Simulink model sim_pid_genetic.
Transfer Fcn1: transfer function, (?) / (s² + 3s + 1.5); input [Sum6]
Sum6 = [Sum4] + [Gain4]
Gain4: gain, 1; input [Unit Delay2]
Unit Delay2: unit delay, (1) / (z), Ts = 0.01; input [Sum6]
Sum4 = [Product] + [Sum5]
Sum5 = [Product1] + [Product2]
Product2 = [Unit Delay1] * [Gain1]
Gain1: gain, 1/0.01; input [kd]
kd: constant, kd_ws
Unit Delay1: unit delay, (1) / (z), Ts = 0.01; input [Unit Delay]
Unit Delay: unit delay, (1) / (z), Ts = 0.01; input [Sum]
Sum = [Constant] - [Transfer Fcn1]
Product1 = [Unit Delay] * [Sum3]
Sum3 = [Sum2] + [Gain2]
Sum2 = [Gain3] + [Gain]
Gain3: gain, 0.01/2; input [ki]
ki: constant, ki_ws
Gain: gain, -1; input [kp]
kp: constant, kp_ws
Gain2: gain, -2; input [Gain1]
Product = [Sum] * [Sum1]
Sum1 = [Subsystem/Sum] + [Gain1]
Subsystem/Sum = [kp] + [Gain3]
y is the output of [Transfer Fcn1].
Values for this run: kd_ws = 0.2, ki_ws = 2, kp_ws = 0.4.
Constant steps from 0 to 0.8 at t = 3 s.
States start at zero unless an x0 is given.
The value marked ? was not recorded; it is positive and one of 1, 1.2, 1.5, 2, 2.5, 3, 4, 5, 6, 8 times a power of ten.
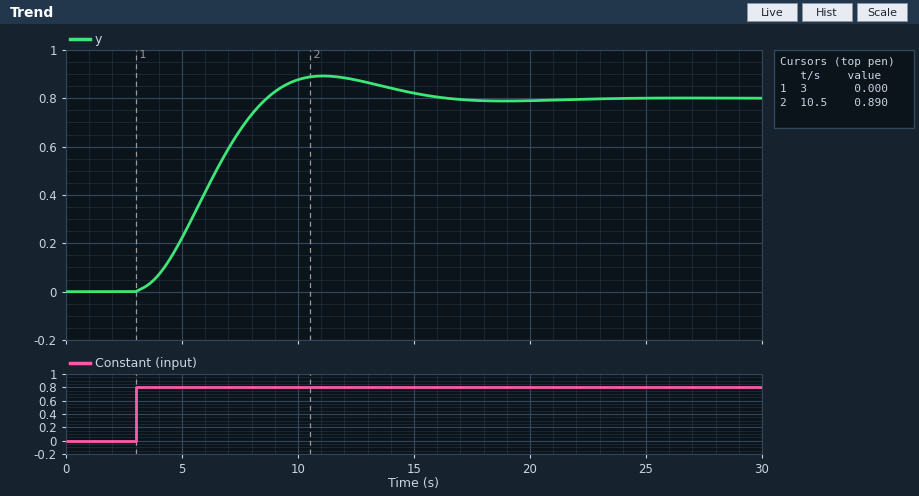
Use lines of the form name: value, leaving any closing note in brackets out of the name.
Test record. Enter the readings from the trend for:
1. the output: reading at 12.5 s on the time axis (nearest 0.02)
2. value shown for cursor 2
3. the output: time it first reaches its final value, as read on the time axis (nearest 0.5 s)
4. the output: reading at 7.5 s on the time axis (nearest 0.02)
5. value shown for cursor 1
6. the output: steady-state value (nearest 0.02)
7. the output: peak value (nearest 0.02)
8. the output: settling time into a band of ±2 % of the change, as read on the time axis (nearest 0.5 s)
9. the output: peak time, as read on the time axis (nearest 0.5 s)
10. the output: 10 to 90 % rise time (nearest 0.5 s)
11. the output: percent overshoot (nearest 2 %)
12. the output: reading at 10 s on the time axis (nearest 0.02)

the output: reading at 12.5 s on the time axis: 0.88
value shown for cursor 2: 0.890
the output: time it first reaches its final value, as read on the time axis: 8.5 s
the output: reading at 7.5 s on the time axis: 0.66
value shown for cursor 1: 0.000
the output: steady-state value: 0.80
the output: peak value: 0.90
the output: settling time into a band of ±2 % of the change, as read on the time axis: 15.5 s
the output: peak time, as read on the time axis: 11.0 s
the output: 10 to 90 % rise time: 4.0 s
the output: percent overshoot: 12 %
the output: reading at 10 s on the time axis: 0.88
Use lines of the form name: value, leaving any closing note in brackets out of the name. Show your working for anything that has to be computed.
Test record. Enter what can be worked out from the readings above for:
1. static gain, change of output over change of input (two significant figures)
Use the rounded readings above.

static gain, change of output over change of input: (0.8 - 0) / (0.8 - 0) = 1.0
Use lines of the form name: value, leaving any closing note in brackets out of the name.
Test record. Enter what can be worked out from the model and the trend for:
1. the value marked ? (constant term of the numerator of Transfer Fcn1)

the value marked ?: 0.3
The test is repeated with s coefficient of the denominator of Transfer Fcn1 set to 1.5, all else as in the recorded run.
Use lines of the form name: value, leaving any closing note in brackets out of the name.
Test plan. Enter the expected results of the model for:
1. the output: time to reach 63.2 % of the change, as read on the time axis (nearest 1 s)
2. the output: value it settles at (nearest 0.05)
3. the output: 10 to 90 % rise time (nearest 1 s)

the output: time to reach 63.2 % of the change, as read on the time axis: 6 s
the output: value it settles at: 0.80
the output: 10 to 90 % rise time: 3 s
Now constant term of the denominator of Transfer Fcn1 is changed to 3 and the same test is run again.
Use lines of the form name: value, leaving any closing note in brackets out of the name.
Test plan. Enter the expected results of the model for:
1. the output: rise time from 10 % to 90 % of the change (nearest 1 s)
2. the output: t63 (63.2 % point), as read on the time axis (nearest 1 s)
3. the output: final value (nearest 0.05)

the output: rise time from 10 % to 90 % of the change: 9 s
the output: t63 (63.2 % point), as read on the time axis: 8 s
the output: final value: 0.80
